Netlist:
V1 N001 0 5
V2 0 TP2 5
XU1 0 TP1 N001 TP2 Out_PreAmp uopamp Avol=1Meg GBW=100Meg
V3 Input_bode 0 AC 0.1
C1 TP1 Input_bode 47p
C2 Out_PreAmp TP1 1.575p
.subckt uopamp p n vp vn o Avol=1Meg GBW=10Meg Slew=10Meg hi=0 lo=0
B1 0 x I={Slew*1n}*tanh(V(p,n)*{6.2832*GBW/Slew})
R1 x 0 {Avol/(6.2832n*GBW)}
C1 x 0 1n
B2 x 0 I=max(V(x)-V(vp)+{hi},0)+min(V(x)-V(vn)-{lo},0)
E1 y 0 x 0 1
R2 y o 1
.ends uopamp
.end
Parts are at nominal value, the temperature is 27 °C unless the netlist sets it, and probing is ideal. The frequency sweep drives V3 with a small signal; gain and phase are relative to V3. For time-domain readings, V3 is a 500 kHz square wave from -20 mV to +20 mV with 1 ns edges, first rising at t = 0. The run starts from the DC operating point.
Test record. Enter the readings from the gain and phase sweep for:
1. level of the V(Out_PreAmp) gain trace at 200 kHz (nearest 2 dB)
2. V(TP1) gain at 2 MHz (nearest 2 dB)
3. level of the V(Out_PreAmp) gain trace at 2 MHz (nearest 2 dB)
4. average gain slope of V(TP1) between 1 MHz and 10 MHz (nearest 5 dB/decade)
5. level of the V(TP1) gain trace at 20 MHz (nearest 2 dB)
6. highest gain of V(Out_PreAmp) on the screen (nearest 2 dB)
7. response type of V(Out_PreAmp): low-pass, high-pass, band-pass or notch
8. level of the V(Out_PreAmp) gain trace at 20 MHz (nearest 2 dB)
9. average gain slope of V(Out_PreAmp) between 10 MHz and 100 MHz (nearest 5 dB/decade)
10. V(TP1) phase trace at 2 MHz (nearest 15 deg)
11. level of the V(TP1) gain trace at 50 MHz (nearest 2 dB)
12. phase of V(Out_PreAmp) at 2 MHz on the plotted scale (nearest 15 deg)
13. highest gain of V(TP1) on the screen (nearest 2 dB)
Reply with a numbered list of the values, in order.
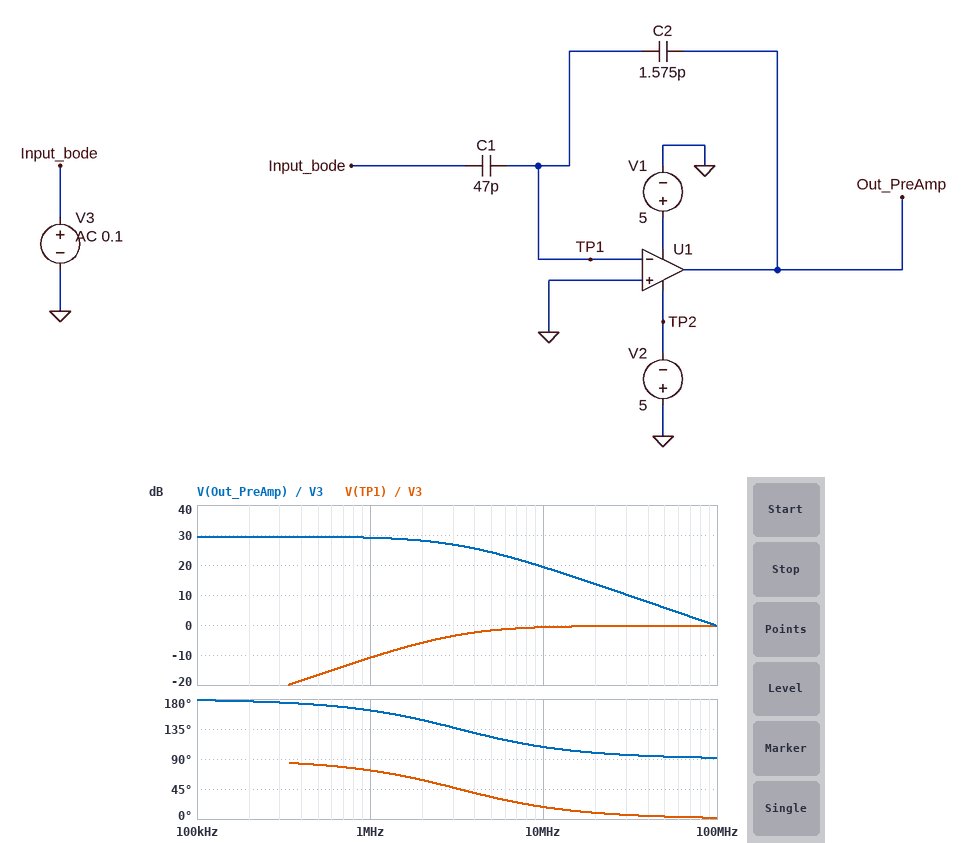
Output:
1. 30 dB
2. -6 dB
3. 28 dB
4. 10 dB/decade
5. 0 dB
6. 30 dB
7. low-pass
8. 14 dB
9. -20 dB/decade
10. 60 deg
11. 0 dB
12. 150 deg
13. 0 dB
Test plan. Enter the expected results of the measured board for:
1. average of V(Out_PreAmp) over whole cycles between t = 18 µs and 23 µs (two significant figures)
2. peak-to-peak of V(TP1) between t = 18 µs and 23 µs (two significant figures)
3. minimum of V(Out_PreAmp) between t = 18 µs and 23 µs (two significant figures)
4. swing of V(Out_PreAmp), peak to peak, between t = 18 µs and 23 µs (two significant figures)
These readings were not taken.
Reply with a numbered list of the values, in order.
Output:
1. -600 mV
2. 77 mV
3. -1.2 V
4. 1.2 V
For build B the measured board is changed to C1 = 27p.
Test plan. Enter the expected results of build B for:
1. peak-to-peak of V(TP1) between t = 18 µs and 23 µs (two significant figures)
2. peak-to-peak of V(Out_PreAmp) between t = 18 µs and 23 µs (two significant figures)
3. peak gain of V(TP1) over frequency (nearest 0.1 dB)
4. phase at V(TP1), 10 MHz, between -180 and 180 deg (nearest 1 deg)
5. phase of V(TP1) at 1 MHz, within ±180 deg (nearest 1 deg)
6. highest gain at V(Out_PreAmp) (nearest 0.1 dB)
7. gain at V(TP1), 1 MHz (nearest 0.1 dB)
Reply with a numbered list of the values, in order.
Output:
1. 75 mV
2. 690 mV
3. -0.5 dB
4. 29 deg
5. 80 deg
6. 24.7 dB
7. -15.5 dB
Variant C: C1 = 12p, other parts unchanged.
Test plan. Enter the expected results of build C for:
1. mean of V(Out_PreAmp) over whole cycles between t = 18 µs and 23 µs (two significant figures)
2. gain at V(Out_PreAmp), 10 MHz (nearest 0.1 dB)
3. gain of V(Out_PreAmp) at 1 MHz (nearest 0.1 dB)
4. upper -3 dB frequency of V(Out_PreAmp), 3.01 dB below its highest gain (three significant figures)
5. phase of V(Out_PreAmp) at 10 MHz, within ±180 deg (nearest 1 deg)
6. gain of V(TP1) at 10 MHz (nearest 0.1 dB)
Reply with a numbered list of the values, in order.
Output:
1. -150 mV
2. 15.2 dB
3. 17.6 dB
4. 11.6 MHz
5. 139 deg
6. -4.8 dB
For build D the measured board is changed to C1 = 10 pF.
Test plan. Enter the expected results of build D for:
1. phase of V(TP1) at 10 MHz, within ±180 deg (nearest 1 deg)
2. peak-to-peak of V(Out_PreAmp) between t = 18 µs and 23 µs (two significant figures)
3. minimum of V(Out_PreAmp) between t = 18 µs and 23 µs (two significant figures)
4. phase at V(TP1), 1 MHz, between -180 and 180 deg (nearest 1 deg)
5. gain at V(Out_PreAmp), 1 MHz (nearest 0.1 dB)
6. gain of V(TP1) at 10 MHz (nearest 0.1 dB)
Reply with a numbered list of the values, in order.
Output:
1. 54 deg
2. 250 mV
3. -250 mV
4. 86 deg
5. 16.0 dB
6. -5.8 dB
